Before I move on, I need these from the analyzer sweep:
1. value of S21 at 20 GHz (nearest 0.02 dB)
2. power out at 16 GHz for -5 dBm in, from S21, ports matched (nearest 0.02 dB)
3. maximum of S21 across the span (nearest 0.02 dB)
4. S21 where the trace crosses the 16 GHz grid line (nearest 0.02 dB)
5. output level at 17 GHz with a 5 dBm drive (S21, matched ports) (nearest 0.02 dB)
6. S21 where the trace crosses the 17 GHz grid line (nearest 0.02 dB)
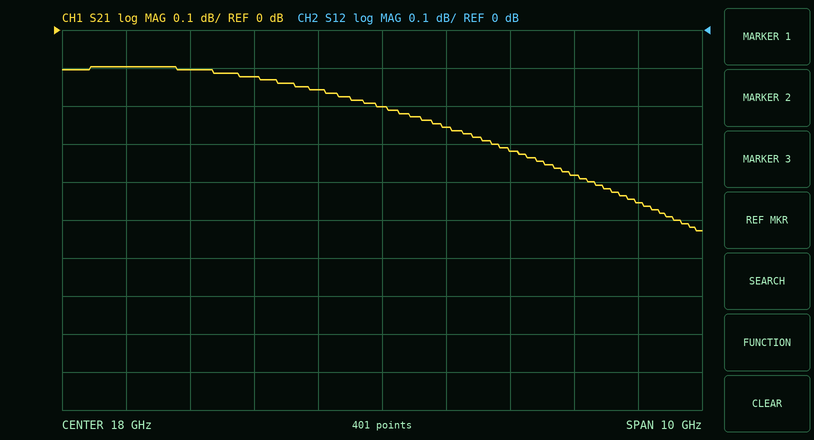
-0.32 dB
-5.12 dBm
-0.10 dB
-0.12 dB
4.84 dBm
-0.16 dB
